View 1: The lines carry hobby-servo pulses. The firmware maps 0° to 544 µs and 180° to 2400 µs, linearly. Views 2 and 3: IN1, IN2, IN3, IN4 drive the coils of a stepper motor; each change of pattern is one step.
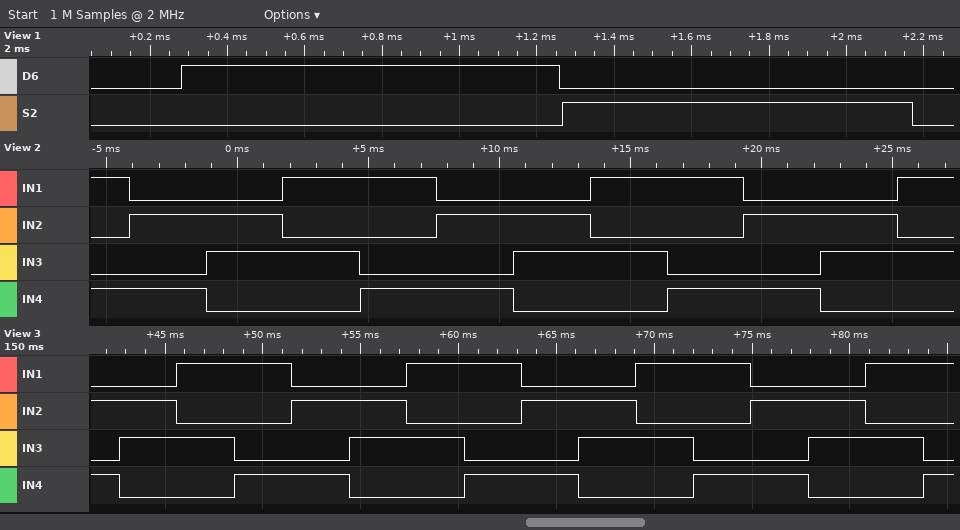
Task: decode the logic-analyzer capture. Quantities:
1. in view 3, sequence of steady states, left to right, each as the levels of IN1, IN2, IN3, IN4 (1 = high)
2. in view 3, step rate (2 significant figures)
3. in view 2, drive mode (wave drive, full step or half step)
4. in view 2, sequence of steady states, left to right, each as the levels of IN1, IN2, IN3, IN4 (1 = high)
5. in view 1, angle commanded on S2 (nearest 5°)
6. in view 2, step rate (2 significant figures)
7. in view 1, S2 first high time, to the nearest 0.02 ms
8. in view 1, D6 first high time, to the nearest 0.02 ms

0101 0110 1010 1001 0101 0110 1010 1001 0101 0110 1010 1001 0101 0110 1010 1001
340 steps/s
full step
1001 0101 0110 1010 1001 0101 0110 1010 1001 0101 0110 1010
35°
340 steps/s
0.90 ms
0.98 ms
